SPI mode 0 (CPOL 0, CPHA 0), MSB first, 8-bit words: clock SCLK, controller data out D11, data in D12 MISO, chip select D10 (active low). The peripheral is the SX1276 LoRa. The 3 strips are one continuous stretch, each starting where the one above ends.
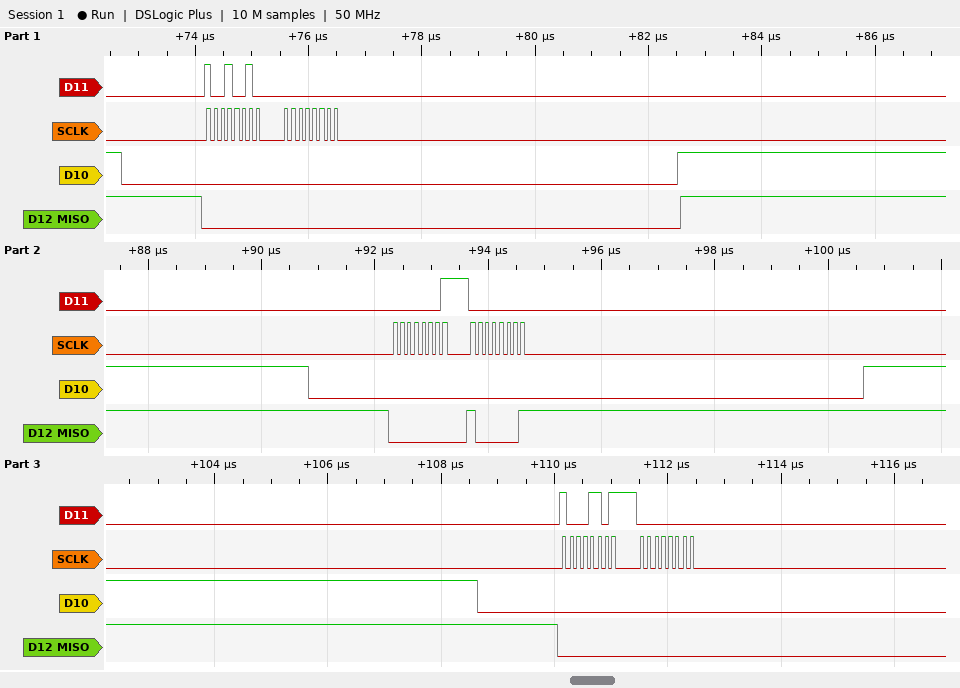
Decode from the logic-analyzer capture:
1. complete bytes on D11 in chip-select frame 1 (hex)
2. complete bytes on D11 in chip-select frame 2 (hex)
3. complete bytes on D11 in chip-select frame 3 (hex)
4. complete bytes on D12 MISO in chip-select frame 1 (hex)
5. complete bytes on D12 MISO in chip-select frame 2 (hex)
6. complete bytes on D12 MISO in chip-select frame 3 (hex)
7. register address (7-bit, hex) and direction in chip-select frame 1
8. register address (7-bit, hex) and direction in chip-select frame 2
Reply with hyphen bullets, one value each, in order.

- 92 00
- 01 00
- 8D 00
- 00 00
- 00 81
- 00 00
- 0x12 write
- 0x01 read
